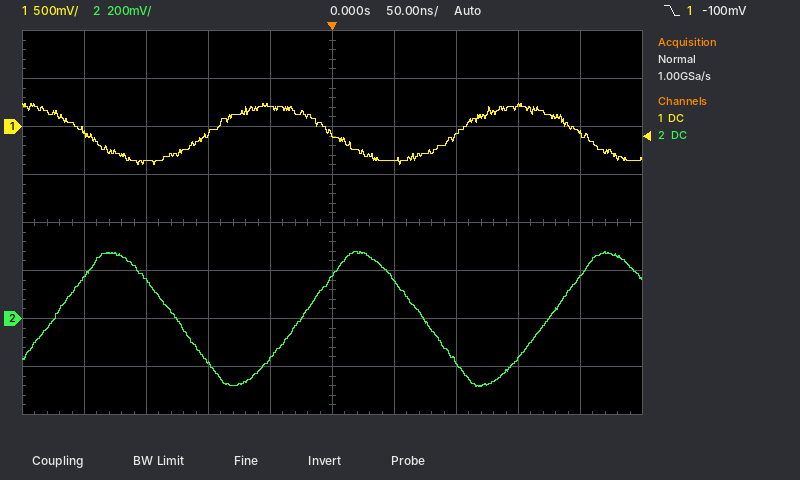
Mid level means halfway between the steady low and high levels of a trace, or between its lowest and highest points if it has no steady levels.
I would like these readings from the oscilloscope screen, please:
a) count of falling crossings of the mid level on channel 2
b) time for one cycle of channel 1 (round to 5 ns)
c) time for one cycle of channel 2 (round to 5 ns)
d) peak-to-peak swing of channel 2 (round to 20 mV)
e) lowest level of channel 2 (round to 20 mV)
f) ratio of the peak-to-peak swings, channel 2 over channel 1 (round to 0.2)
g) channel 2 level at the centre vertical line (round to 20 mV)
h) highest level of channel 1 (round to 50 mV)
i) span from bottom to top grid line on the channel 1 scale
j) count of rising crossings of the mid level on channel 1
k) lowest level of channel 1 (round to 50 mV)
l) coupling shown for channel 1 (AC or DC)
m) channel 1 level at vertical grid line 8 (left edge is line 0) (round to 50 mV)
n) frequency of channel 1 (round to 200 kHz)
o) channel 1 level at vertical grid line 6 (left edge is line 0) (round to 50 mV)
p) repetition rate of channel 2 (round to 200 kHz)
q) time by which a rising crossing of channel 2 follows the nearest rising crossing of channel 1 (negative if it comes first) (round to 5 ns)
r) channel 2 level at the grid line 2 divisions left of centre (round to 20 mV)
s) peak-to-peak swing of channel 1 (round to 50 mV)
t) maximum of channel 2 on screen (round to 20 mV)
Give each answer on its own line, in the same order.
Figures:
2
200 ns
200 ns
560 mV
-280 mV
0.8
180 mV
250 mV
4 V
2
-400 mV
DC
200 mV
5.0 MHz
-350 mV
5.0 MHz
+75 ns
-180 mV
650 mV
280 mV
